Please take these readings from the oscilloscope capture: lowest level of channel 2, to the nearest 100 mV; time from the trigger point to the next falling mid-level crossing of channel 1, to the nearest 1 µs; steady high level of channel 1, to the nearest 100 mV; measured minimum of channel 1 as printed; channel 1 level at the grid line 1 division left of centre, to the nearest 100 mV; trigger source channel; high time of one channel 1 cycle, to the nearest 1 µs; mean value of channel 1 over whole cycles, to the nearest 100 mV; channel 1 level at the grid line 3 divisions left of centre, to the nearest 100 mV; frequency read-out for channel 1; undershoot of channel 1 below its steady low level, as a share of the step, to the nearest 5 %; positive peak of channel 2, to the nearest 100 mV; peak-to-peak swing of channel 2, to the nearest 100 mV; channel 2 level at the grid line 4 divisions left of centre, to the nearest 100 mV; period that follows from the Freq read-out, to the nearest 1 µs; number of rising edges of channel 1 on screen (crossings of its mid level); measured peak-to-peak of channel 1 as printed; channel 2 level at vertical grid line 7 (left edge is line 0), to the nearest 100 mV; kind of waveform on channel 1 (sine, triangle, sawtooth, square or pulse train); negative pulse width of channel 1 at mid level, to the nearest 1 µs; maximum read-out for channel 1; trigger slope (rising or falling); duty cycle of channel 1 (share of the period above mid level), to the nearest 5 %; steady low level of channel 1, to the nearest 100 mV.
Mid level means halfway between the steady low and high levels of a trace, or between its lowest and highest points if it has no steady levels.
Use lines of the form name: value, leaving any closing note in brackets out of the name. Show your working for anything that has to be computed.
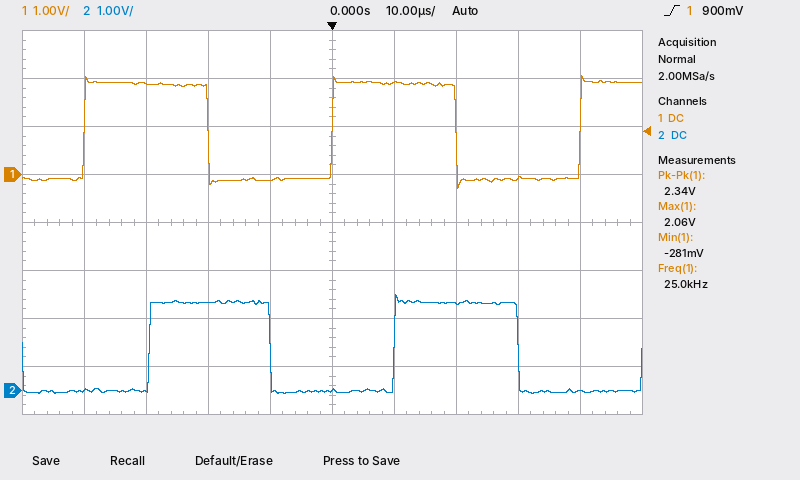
lowest level of channel 2, to the nearest 100 mV: -100 mV
time from the trigger point to the next falling mid-level crossing of channel 1, to the nearest 1 µs: 20 µs
steady high level of channel 1, to the nearest 100 mV: 1.9 V
measured minimum of channel 1 as printed: -281 mV
channel 1 level at the grid line 1 division left of centre, to the nearest 100 mV: -100 mV
trigger source channel: channel 1
high time of one channel 1 cycle, to the nearest 1 µs: 20 µs
mean value of channel 1 over whole cycles, to the nearest 100 mV: -100 mV + 0.5 × (1.9 V − (-100 mV)) ≈ 900 mV
channel 1 level at the grid line 3 divisions left of centre, to the nearest 100 mV: 1.9 V
frequency read-out for channel 1: 25.0 kHz
undershoot of channel 1 below its steady low level, as a share of the step, to the nearest 5 %: 10 %
positive peak of channel 2, to the nearest 100 mV: 2.0 V
peak-to-peak swing of channel 2, to the nearest 100 mV: 2.0 V − (-100 mV) = 2.1 V
channel 2 level at the grid line 4 divisions left of centre, to the nearest 100 mV: 0.0 V
period that follows from the Freq read-out, to the nearest 1 µs: 1 / 25.0 kHz ≈ 40 µs
number of rising edges of channel 1 on screen: 3
measured peak-to-peak of channel 1 as printed: 2.34 V
channel 2 level at vertical grid line 7 (left edge is line 0), to the nearest 100 mV: 1.8 V
kind of waveform on channel 1: square
negative pulse width of channel 1 at mid level, to the nearest 1 µs: 20 µs
maximum read-out for channel 1: 2.06 V
trigger slope: rising
duty cycle of channel 1 (share of the period above mid level), to the nearest 5 %: 50 %
steady low level of channel 1, to the nearest 100 mV: -100 mV
